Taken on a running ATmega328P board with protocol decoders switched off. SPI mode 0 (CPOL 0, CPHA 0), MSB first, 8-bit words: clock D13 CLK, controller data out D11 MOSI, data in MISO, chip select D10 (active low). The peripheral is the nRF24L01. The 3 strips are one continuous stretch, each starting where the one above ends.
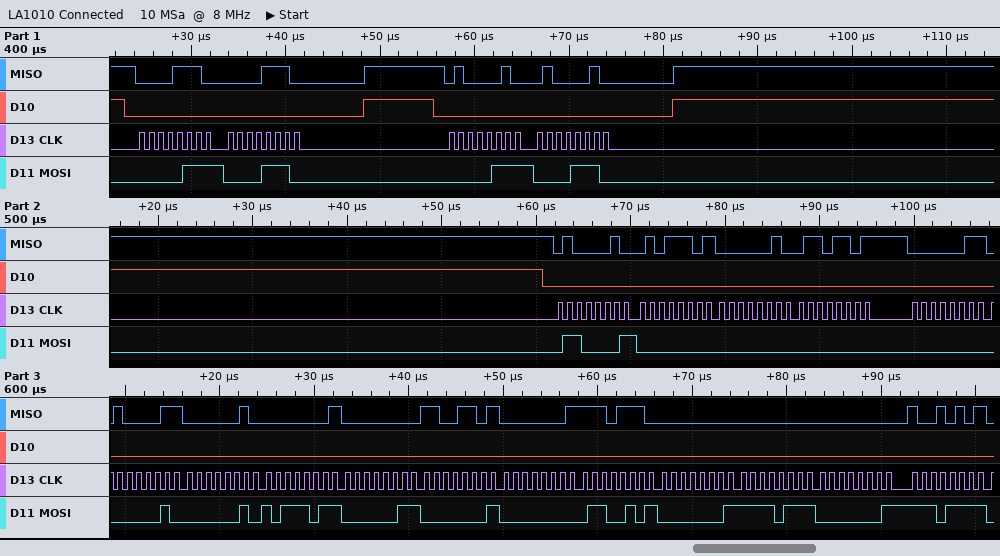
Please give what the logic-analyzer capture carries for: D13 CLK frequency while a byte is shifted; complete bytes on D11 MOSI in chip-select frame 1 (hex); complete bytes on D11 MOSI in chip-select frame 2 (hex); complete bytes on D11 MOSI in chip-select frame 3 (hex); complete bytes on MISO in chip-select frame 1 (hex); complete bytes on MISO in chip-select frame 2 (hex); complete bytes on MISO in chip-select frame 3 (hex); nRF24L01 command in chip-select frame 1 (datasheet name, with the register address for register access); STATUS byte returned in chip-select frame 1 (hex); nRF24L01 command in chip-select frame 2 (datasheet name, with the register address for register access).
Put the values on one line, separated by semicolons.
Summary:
1 MHz; 07 0E; 07 0E; 61 00 00 00 00 02 02 BB 03 01 00 65 01 F7 01 EF; 0E 0E; 42 42; 42 5D 02 6D 03 43 02 01 00 CD 01 EE 00 00 00 95; R_REGISTER 0x07; 0x0E; R_REGISTER 0x07
